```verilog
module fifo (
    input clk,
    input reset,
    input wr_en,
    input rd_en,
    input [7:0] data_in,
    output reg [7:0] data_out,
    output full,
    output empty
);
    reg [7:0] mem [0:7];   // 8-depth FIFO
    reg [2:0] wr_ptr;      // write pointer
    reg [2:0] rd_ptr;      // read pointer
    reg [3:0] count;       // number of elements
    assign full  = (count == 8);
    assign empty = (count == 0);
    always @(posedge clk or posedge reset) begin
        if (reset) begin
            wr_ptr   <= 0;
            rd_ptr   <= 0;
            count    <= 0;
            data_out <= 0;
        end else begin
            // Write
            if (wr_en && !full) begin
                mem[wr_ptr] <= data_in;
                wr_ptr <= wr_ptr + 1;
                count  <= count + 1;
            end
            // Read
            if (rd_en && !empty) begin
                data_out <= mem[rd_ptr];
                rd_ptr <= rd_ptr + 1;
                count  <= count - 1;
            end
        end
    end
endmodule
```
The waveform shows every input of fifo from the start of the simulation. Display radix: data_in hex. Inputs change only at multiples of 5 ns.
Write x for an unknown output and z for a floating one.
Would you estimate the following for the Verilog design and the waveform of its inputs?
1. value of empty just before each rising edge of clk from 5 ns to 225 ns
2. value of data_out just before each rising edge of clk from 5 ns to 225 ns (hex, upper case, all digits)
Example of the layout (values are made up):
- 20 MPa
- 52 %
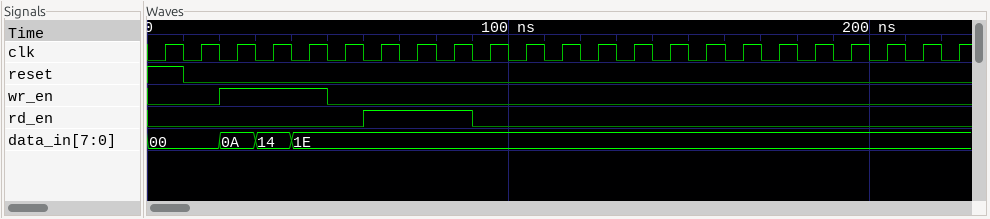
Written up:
- 1 1 1 0 0 0 0 0 0 1 1 1 1 1 1 1 1 1 1 1 1 1 1
- 00, 00, 00, 00, 00, 00, 00, 0A, 14, 1E, 1E, 1E, 1E, 1E, 1E, 1E, 1E, 1E, 1E, 1E, 1E, 1E, 1E
